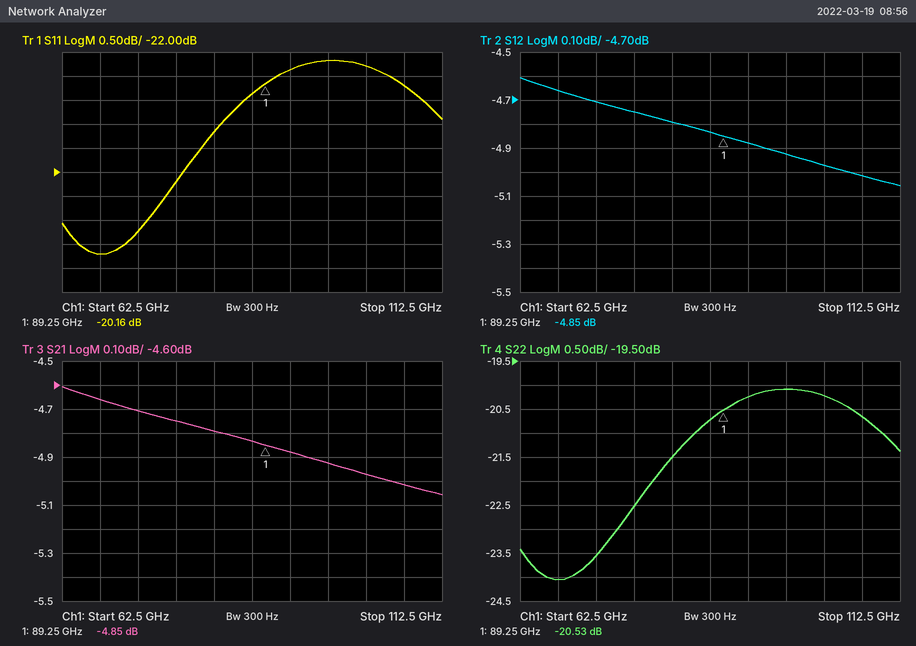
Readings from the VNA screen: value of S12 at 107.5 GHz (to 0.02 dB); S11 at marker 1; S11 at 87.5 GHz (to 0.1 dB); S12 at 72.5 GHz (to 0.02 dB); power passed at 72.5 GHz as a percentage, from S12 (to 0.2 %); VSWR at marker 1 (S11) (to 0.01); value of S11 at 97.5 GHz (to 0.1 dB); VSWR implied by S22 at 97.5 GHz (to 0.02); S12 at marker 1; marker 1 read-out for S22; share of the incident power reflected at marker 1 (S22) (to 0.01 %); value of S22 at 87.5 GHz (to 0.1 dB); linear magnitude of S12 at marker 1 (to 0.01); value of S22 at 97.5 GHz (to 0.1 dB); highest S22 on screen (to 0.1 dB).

-5.02 dB
-20.16 dB
-20.4 dB
-4.70 dB
33.8 %
1.22
-19.7 dB
1.22
-4.85 dB
-20.53 dB
0.89 %
-20.7 dB
0.57
-20.1 dB
-20.1 dB
